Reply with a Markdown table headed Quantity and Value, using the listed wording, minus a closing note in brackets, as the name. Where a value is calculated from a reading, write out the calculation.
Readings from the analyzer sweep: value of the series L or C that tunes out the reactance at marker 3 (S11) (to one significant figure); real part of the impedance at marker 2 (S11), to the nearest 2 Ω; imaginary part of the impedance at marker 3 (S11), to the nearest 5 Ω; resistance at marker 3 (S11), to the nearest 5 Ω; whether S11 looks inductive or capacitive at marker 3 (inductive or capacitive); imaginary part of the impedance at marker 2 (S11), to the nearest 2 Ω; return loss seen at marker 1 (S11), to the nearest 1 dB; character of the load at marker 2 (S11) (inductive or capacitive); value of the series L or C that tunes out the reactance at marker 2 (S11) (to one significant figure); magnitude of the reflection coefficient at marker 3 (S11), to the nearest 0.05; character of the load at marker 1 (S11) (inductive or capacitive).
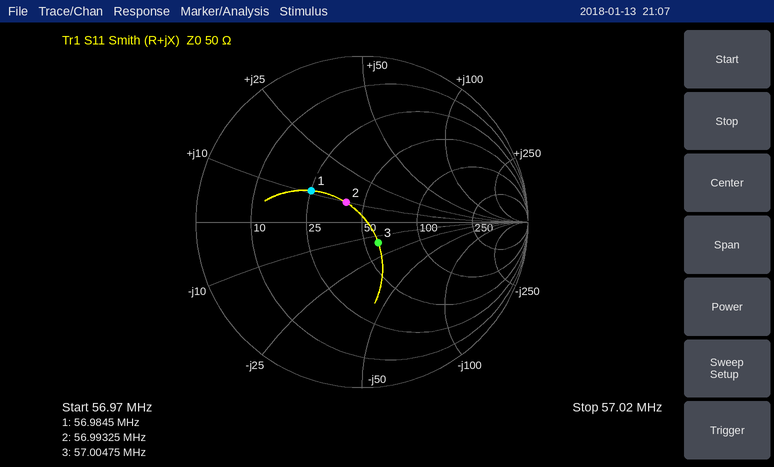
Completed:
| Quantity | Value |
|---|---|
| value of the series L or C that tunes out the reactance at marker 3 (S11) | L = 15 Ω/(2π × 57.00475 MHz) ≈ 41.9 nH, so 40 nH to one significant figure |
| real part of the impedance at marker 2 (S11), to the nearest 2 Ω | 40 Ω |
| imaginary part of the impedance at marker 3 (S11), to the nearest 5 Ω | -15 Ω |
| resistance at marker 3 (S11), to the nearest 5 Ω | 60 Ω |
| whether S11 looks inductive or capacitive at marker 3 | capacitive |
| imaginary part of the impedance at marker 2 (S11), to the nearest 2 Ω | +10 Ω |
| return loss seen at marker 1 (S11), to the nearest 1 dB | 9 dB |
| character of the load at marker 2 (S11) | inductive |
| value of the series L or C that tunes out the reactance at marker 2 (S11) | C = 1/(2π × 56.99325 MHz × 10 Ω) ≈ 279 pF, so 300 pF to one significant figure |
| magnitude of the reflection coefficient at marker 3 (S11), to the nearest 0.05 | 0.15 |
| character of the load at marker 1 (S11) | inductive |
